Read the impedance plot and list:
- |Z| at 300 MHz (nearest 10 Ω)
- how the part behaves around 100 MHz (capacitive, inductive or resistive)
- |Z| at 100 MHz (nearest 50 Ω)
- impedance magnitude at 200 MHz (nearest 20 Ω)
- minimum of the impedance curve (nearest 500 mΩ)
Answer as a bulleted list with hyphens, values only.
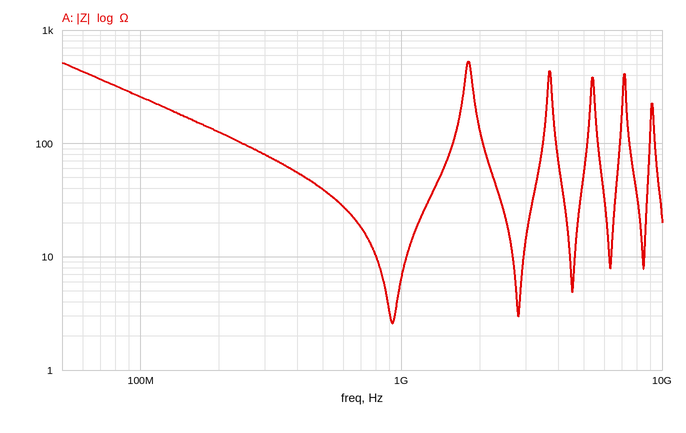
- 80 Ω
- capacitive
- 250 Ω
- 120 Ω
- 2.5 Ω
